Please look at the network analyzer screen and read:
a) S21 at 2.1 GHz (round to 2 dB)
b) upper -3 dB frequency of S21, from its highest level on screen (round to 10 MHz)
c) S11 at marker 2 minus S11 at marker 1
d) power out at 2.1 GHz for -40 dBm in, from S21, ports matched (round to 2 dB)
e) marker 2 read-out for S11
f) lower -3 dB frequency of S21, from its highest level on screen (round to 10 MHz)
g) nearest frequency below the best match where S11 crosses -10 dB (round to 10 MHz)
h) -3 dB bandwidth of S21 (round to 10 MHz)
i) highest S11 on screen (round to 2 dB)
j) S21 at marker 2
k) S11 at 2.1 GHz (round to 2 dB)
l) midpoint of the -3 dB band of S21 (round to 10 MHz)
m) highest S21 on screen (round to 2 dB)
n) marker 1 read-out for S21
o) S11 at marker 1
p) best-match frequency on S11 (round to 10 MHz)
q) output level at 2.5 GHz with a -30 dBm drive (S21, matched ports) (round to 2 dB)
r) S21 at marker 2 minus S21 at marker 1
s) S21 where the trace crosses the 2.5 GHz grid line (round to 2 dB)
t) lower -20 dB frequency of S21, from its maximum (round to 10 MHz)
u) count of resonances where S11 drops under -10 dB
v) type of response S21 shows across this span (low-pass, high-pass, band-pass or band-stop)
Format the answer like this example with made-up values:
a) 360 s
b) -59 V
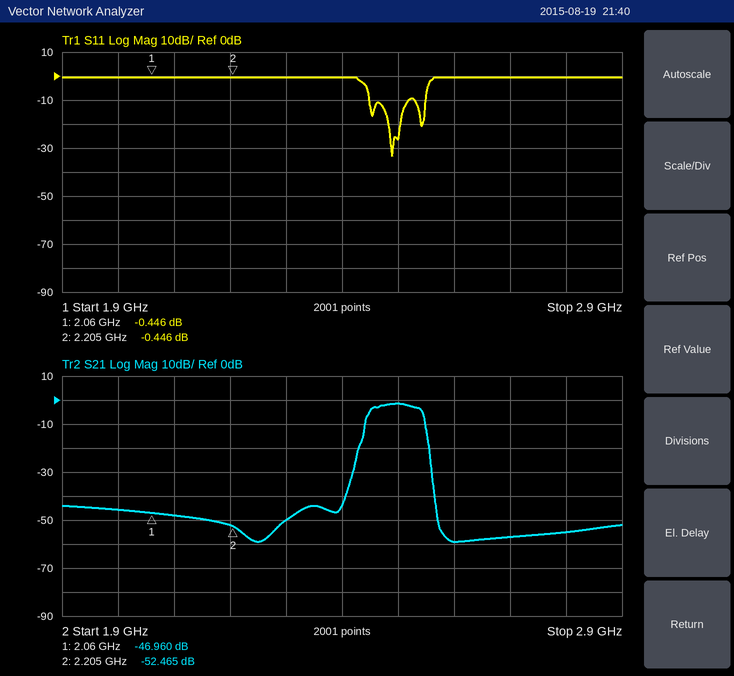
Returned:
a) -48 dB
b) 2.54 GHz
c) 0.000 dB
d) -88 dBm
e) -0.446 dB
f) 2.45 GHz
g) 2.45 GHz
h) 90 MHz
i) 0 dB
j) -52.465 dB
k) 0 dB
l) 2.50 GHz
m) -2 dB
n) -46.960 dB
o) -0.446 dB
p) 2.49 GHz
q) -32 dBm
r) -5.505 dB
s) -2 dB
t) 2.43 GHz
u) 3
v) band-pass
